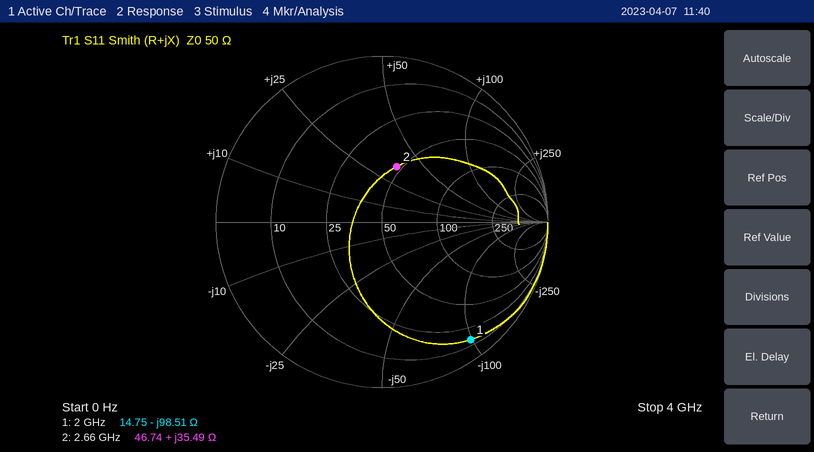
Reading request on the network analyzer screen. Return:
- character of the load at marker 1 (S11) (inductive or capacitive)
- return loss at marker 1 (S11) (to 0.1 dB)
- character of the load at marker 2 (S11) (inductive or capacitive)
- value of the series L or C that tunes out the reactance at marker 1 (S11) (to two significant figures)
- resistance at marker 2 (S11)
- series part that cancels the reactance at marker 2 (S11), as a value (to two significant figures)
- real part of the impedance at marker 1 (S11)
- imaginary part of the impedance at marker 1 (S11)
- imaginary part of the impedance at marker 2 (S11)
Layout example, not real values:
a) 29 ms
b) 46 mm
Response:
a) capacitive
b) 1.0 dB
c) inductive
d) 7.8 nH
e) 46.74 Ω
f) 1.7 pF
g) 14.75 Ω
h) -98.51 Ω
i) +35.49 Ω
